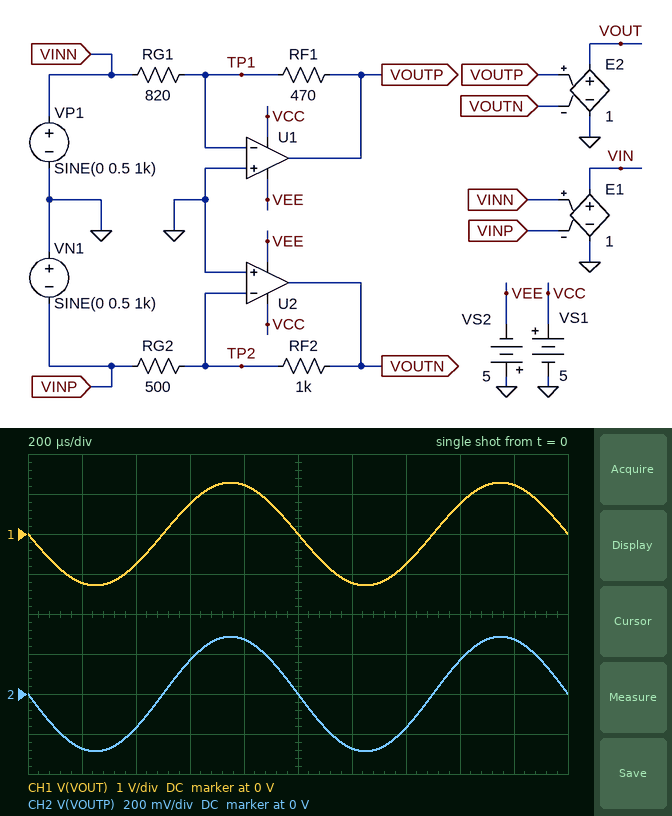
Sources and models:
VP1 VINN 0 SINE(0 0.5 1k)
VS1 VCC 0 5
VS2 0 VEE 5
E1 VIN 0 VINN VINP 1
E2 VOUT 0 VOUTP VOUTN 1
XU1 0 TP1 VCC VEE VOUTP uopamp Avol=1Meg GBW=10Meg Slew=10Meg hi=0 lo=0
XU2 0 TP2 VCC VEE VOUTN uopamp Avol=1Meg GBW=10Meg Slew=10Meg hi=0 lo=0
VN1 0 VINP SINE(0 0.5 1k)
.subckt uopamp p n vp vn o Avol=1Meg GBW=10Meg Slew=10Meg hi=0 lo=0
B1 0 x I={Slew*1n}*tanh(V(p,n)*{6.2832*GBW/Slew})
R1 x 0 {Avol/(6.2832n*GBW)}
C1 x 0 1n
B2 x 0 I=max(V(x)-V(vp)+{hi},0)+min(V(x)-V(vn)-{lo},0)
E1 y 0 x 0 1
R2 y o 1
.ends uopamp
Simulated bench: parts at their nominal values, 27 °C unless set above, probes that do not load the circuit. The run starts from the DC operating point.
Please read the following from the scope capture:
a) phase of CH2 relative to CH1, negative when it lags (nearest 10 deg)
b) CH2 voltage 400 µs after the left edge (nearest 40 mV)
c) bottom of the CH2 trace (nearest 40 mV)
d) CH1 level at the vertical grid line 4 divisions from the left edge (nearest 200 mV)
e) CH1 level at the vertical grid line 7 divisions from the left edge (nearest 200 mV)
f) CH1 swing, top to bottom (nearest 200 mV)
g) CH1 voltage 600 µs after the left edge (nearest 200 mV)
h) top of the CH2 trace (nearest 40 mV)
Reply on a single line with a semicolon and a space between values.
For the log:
0 deg; -160 mV; -280 mV; 1.2 V; -800 mV; 2.6 V; 800 mV; 280 mV
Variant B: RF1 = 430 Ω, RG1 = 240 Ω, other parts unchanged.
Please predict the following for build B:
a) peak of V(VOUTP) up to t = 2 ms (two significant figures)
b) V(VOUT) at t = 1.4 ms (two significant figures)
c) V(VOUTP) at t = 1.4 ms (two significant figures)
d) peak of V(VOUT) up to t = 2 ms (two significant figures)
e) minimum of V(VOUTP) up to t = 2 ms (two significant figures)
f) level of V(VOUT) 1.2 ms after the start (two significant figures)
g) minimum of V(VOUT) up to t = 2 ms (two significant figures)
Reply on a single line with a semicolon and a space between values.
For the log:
900 mV; -1.1 V; -530 mV; 1.9 V; -900 mV; -1.8 V; -1.9 V
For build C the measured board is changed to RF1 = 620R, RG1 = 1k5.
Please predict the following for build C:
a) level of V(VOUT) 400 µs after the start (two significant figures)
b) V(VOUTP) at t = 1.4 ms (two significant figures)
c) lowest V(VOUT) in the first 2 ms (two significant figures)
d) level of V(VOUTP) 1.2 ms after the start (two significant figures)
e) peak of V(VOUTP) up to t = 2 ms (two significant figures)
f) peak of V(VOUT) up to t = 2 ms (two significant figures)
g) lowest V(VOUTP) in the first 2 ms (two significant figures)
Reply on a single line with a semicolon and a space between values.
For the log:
-710 mV; -120 mV; -1.2 V; -200 mV; 210 mV; 1.2 V; -210 mV
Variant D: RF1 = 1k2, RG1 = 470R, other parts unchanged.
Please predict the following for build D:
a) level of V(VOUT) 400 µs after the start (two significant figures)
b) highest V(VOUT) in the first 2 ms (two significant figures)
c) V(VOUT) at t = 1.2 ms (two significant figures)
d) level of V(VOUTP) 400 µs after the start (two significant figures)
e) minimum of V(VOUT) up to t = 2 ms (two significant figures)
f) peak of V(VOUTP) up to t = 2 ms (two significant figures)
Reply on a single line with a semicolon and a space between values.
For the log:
-1.3 V; 2.3 V; -2.2 V; -750 mV; -2.3 V; 1.3 V
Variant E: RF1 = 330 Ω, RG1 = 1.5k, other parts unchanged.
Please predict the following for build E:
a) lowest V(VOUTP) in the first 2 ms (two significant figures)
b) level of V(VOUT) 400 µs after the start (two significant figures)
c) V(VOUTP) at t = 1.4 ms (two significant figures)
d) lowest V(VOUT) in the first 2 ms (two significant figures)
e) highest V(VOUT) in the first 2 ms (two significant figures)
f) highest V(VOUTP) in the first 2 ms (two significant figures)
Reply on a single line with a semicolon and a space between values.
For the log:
-110 mV; -650 mV; -65 mV; -1.1 V; 1.1 V; 110 mV
